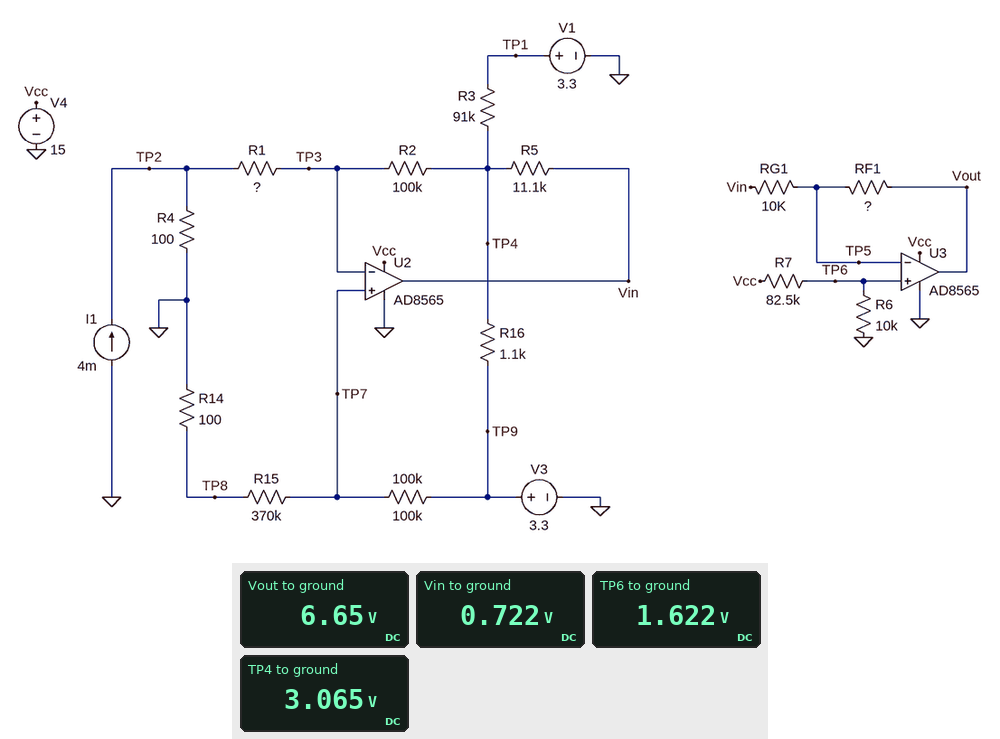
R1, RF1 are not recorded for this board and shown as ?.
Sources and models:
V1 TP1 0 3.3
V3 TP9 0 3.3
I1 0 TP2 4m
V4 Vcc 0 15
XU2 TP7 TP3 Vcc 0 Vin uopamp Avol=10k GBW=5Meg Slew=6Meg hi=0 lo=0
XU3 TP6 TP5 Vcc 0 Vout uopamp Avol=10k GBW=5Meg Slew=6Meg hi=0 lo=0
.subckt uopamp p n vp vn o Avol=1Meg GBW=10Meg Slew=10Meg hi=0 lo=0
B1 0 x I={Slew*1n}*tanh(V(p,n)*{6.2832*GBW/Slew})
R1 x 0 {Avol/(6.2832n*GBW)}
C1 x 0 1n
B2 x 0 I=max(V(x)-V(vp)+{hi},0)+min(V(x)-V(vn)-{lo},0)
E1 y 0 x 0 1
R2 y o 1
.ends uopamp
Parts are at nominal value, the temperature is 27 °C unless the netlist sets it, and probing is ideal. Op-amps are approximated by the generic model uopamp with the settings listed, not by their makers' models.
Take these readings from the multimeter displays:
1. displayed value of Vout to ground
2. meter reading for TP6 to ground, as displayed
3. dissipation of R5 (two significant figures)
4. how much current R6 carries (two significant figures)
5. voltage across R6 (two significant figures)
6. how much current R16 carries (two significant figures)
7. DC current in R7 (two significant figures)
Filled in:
6.65 V
1.622 V
490 µW
160 µA
1.6 V
210 µA
160 µA
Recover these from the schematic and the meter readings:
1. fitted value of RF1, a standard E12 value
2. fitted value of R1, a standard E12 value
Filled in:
56 kΩ
470 kΩ
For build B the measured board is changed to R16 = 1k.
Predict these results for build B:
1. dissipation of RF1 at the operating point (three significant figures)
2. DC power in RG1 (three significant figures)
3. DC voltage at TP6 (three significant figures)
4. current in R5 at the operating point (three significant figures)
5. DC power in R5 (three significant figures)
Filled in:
721 µW
129 µW
1.62 V
232 µA
599 µW
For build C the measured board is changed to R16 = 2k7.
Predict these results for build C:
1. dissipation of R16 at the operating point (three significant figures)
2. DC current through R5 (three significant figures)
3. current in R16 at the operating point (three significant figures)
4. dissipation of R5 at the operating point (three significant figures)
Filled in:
20.4 µW
84.8 µA
86.9 µA
79.9 µW
